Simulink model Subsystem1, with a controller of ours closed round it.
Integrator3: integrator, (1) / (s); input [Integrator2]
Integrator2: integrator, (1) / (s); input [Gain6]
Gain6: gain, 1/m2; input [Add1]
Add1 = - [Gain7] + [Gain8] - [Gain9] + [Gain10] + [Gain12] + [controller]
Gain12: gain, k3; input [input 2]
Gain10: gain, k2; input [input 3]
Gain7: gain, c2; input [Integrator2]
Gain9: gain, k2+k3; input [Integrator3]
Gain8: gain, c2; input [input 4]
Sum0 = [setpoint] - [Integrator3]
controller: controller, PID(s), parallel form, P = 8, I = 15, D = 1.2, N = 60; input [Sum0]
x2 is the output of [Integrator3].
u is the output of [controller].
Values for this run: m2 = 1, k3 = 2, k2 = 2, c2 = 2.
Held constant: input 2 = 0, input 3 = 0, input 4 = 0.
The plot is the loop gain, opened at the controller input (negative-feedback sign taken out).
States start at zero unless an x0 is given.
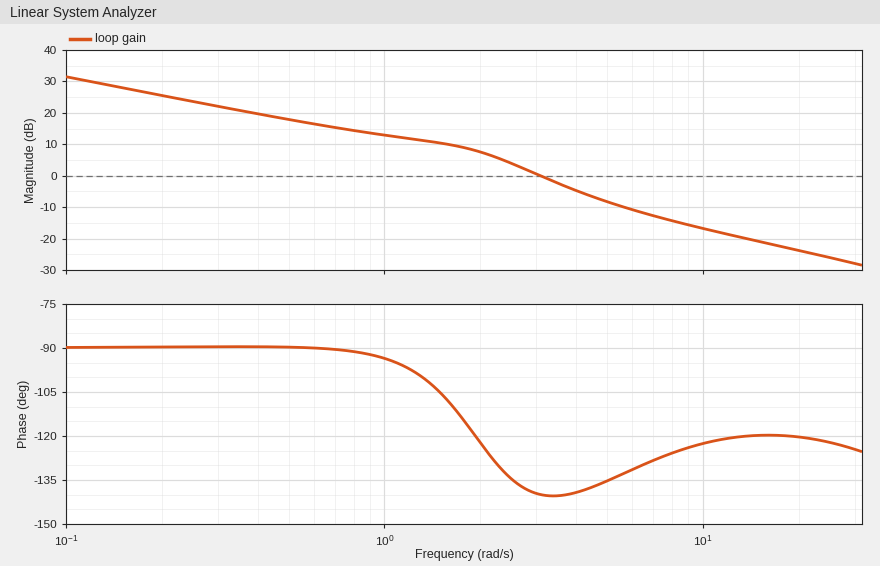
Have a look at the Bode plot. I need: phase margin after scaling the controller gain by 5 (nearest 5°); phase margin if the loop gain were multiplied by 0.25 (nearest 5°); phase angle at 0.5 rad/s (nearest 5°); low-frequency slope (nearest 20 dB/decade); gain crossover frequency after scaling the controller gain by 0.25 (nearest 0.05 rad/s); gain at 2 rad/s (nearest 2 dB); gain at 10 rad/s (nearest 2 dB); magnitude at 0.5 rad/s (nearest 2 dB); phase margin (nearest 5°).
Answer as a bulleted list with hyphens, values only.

- 55°
- 85°
- -90°
- -20 dB/decade
- 1.15 rad/s
- 8 dB
- -16 dB
- 18 dB
- 40°
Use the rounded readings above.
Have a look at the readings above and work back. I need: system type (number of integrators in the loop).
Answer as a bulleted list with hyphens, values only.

- 1
